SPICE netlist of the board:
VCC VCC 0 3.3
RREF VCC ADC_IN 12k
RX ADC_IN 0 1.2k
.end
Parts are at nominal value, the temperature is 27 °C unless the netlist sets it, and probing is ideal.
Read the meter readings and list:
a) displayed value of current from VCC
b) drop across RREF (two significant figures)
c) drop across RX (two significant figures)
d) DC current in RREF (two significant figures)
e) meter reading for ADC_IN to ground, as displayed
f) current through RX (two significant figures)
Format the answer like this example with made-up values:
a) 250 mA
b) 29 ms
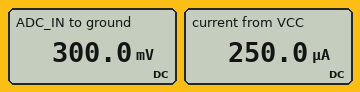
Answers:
a) 250.0 µA
b) 3.0 V
c) 300 mV
d) 250 µA
e) 300.0 mV
f) 250 µA
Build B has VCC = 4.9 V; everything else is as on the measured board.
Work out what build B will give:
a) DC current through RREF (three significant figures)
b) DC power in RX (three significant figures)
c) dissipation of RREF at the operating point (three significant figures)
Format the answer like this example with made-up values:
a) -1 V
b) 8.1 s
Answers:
a) 371 µA
b) 165 µW
c) 1.65 mW
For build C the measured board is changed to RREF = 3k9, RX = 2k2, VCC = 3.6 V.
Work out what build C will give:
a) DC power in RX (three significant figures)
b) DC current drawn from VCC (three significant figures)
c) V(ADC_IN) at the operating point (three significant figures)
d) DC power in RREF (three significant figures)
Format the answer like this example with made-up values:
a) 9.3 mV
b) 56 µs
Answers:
a) 766 µW
b) 590 µA
c) 1.30 V
d) 1.36 mW
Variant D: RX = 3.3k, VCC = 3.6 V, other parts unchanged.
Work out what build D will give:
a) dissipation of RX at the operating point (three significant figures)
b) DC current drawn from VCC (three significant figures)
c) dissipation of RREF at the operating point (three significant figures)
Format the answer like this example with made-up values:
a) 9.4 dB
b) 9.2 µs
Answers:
a) 183 µW
b) 235 µA
c) 664 µW
